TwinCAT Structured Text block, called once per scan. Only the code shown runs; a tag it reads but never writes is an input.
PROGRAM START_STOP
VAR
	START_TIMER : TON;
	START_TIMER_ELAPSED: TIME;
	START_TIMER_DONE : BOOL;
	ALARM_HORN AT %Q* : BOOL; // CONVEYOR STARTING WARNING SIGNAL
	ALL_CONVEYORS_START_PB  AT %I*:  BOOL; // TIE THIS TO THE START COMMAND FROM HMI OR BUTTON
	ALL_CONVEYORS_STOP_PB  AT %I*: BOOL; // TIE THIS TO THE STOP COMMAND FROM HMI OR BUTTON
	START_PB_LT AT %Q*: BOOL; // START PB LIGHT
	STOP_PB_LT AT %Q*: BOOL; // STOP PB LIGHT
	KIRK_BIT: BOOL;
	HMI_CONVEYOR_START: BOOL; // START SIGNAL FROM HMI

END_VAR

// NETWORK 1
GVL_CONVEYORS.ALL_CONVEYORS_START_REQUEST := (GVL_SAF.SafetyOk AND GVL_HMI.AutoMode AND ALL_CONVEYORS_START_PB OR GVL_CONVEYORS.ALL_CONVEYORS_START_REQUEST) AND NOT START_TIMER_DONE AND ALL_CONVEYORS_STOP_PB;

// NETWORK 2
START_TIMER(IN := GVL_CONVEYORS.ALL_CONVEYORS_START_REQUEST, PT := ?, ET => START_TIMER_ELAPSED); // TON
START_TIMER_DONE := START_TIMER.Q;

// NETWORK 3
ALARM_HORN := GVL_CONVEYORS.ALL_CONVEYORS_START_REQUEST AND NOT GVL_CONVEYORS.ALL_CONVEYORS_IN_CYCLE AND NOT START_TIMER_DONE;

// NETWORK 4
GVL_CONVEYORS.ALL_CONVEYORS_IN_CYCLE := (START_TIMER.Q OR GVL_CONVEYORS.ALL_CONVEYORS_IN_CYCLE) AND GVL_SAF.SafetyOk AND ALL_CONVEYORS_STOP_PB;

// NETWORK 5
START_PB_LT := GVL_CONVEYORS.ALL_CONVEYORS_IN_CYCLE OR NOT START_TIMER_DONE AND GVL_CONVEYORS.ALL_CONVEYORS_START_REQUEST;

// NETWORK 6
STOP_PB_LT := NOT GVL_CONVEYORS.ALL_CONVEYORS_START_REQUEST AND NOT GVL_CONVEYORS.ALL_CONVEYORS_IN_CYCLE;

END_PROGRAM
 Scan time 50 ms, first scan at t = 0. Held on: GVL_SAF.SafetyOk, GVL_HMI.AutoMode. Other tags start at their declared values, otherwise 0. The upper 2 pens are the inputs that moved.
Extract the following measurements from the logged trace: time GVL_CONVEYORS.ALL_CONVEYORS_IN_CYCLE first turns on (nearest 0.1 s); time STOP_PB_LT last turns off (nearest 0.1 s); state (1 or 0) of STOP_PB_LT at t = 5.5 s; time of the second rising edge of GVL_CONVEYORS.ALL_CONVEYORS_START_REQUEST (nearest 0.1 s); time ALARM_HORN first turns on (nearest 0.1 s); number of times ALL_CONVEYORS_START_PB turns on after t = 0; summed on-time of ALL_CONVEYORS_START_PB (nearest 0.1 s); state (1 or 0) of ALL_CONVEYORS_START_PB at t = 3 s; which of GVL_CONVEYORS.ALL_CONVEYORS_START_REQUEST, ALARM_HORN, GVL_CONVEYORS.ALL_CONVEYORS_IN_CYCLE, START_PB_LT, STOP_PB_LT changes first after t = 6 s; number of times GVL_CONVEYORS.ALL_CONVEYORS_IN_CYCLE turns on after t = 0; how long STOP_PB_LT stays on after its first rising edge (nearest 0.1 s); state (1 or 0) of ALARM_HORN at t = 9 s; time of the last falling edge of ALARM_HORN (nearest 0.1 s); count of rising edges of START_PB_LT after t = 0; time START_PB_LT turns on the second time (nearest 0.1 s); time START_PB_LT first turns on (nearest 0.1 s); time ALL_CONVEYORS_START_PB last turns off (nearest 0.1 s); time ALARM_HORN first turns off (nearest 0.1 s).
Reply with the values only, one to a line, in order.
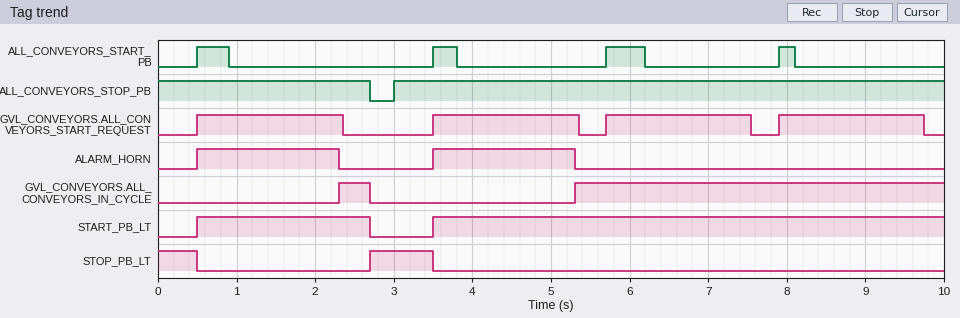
2.3 s
3.5 s
0
3.5 s
0.5 s
4
1.4 s
0
GVL_CONVEYORS.ALL_CONVEYORS_START_REQUEST
2
0.8 s
0
5.3 s
2
3.5 s
0.5 s
8.1 s
2.3 s
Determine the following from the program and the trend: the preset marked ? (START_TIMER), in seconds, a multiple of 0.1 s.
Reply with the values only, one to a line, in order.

1.8 s
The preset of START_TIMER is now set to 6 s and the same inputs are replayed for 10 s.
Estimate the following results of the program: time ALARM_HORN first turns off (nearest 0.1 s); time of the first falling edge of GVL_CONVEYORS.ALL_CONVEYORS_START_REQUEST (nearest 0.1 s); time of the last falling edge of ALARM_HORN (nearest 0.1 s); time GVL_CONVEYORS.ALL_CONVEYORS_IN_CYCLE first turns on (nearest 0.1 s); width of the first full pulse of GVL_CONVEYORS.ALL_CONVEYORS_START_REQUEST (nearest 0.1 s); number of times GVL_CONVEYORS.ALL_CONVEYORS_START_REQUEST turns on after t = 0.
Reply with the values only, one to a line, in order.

2.7 s
2.7 s
9.5 s
9.5 s
2.2 s
2
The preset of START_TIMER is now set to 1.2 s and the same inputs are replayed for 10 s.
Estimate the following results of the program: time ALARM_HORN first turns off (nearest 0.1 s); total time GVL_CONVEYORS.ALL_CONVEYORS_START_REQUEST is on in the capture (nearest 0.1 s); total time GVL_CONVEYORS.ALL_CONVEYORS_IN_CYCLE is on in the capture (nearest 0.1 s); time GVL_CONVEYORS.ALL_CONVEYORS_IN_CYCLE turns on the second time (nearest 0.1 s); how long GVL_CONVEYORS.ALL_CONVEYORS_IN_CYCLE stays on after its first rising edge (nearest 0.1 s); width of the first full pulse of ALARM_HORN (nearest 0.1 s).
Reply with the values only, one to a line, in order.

1.7 s
5.0 s
6.3 s
4.7 s
1.0 s
1.2 s
